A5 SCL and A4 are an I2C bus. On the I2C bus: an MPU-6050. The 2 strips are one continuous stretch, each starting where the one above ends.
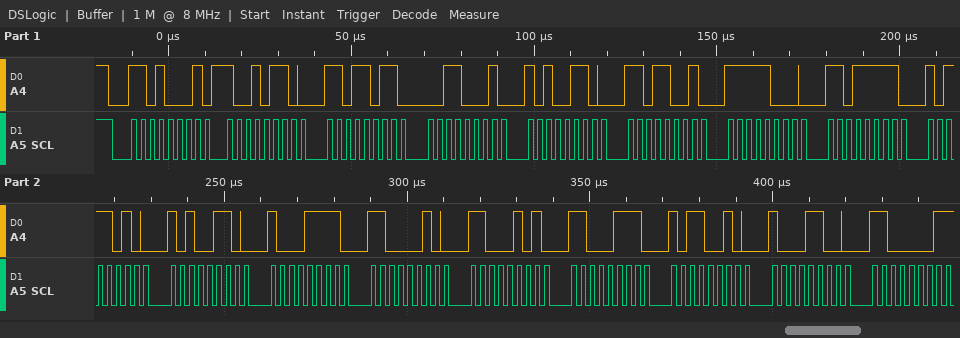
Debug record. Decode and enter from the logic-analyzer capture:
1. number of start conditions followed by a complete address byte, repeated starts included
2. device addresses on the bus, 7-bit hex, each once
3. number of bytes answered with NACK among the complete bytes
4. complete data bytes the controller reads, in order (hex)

1
0x68
1
96 DB 31 A6 D9 F8 DF BA A6 8F C2 C5 C7 B2 8C C1
